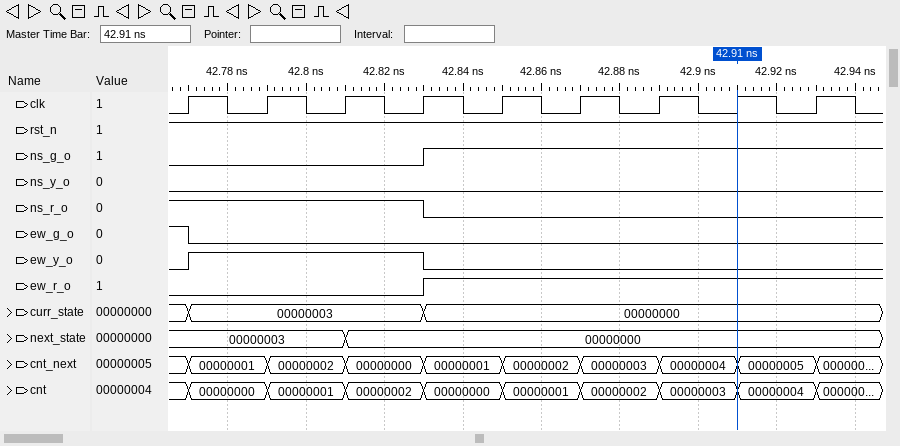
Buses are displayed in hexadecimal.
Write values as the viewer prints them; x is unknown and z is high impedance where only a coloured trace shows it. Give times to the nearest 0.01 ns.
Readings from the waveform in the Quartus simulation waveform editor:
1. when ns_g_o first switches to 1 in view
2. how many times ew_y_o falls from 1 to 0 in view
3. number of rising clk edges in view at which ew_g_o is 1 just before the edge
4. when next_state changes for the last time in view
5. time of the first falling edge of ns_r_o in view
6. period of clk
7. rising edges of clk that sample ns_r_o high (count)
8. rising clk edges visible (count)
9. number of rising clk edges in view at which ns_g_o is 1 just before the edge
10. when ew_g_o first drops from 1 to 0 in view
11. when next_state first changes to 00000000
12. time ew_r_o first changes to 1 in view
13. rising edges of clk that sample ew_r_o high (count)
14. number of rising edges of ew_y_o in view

42.83 ns
1
1
42.81 ns
42.83 ns
0.02 ns
4
9
5
42.77 ns
42.81 ns
42.83 ns
5
1
